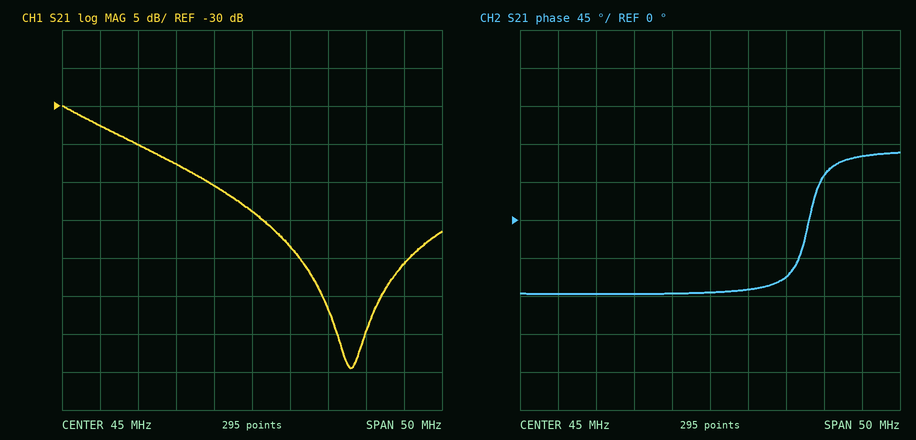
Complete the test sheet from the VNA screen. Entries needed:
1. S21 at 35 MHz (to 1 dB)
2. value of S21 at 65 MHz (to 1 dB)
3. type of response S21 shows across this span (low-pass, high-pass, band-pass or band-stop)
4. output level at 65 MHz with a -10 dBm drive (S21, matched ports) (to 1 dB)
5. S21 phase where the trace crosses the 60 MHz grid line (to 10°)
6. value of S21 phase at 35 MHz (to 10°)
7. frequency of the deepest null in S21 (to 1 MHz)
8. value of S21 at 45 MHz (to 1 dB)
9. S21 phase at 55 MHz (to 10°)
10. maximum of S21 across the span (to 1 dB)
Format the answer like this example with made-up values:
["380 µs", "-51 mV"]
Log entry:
["-38 dB", "-51 dB", "low-pass", "-61 dBm", "50°", "-90°", "58 MHz", "-44 dB", "-70°", "-30 dB"]
